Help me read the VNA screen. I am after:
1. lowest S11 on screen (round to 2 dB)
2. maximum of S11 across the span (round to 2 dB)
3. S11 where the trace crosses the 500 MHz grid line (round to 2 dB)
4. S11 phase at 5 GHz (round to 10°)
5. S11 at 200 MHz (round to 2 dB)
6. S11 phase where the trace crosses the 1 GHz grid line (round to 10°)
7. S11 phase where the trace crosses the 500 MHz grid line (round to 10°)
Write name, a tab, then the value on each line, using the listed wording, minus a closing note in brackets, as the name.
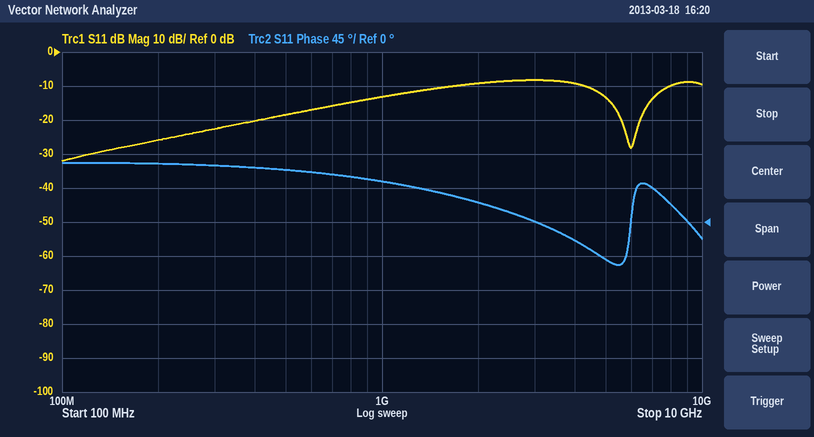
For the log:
lowest S11 on screen	-32 dB
maximum of S11 across the span	-8 dB
S11 where the trace crosses the 500 MHz grid line	-18 dB
S11 phase at 5 GHz	-50°
S11 at 200 MHz	-26 dB
S11 phase where the trace crosses the 1 GHz grid line	50°
S11 phase where the trace crosses the 500 MHz grid line	70°
